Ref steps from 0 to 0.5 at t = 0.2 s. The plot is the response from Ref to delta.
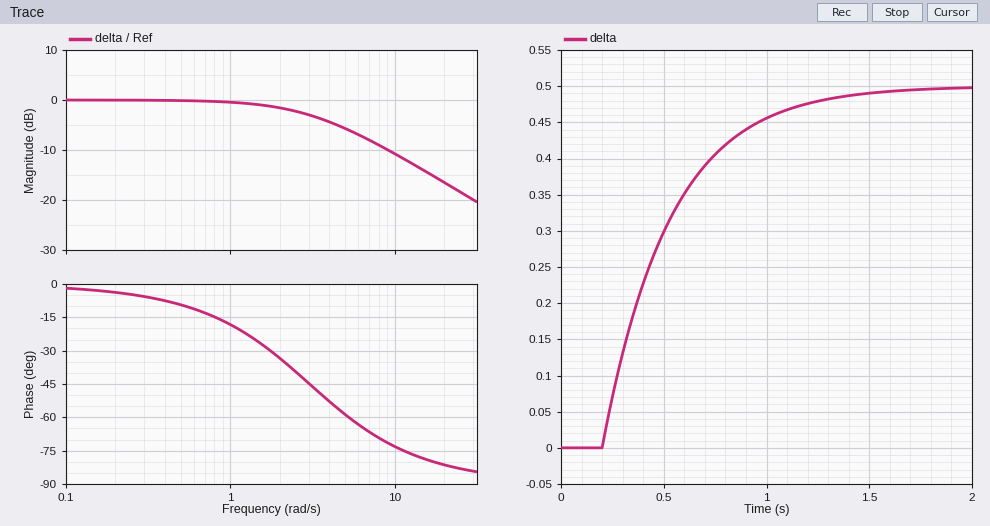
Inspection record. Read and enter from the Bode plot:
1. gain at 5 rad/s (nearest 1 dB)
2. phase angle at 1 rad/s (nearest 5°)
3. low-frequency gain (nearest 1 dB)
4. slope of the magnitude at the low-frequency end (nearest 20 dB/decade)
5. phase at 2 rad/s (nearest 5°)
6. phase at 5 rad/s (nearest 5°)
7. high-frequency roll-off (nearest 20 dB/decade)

-6 dB
-20°
0 dB
0 dB/decade
-35°
-60°
-20 dB/decade
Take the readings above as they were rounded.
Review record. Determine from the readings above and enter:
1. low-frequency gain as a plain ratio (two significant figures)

1.0
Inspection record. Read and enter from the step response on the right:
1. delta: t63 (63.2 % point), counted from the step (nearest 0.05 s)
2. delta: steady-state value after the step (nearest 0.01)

0.35 s
0.50
